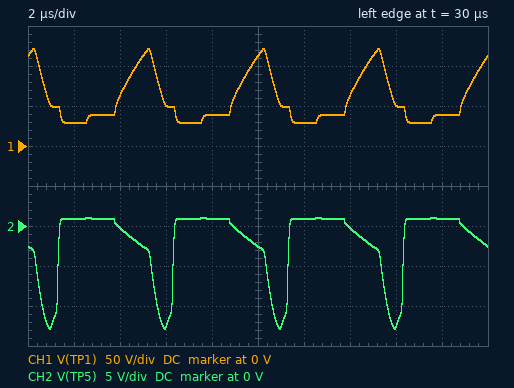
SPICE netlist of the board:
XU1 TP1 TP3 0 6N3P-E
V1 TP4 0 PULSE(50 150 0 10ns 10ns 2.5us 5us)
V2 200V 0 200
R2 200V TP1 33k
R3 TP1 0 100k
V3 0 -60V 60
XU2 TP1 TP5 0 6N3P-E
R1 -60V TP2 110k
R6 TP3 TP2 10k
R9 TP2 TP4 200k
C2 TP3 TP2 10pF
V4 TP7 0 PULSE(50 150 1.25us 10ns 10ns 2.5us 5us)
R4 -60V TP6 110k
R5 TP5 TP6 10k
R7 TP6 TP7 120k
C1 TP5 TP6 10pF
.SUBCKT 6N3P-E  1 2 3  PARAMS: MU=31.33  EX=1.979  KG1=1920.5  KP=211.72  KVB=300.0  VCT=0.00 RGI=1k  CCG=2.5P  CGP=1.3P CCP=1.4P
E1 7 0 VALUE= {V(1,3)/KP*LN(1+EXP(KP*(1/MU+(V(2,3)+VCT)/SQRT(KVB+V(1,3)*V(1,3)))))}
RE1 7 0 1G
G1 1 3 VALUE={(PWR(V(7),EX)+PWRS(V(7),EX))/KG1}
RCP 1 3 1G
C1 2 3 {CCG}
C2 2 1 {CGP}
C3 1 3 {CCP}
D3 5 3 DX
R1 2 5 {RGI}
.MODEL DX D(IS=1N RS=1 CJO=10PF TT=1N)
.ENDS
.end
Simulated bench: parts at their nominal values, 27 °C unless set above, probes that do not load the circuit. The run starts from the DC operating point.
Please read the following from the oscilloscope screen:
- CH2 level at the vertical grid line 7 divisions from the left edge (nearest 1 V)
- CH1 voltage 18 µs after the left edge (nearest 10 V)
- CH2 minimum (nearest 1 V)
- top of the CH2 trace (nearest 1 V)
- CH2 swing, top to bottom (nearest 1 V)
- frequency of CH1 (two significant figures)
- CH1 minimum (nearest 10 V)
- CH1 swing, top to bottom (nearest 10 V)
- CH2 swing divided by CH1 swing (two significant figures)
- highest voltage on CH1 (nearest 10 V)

0 V
40 V
-13 V
1 V
14 V
200 kHz
30 V
90 V
0.15
120 V
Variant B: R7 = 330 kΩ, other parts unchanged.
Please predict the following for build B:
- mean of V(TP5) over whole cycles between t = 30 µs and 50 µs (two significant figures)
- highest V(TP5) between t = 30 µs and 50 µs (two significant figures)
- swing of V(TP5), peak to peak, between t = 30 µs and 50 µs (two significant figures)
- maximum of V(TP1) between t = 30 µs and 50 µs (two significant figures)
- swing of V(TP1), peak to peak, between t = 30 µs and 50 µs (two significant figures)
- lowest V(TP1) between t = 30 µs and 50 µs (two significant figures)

-20 V
-2.4 V
40 V
150 V
100 V
48 V
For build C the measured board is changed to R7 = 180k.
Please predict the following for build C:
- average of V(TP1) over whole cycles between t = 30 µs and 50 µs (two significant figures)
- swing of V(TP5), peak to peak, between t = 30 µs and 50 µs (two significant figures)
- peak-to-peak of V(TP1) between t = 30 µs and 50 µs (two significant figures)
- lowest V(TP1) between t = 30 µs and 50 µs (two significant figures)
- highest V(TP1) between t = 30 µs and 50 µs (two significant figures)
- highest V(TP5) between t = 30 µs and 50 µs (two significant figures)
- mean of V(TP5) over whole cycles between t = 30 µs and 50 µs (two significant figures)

76 V
27 V
120 V
33 V
150 V
690 mV
-6.9 V
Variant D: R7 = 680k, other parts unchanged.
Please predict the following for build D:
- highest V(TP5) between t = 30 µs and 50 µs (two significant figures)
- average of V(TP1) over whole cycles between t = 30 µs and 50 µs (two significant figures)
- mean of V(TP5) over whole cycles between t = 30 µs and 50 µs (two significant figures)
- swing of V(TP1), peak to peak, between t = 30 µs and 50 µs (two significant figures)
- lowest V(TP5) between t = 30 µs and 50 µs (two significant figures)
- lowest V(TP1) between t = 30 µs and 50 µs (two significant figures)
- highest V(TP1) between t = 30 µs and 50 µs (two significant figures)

-20 V
110 V
-38 V
100 V
-56 V
48 V
150 V
